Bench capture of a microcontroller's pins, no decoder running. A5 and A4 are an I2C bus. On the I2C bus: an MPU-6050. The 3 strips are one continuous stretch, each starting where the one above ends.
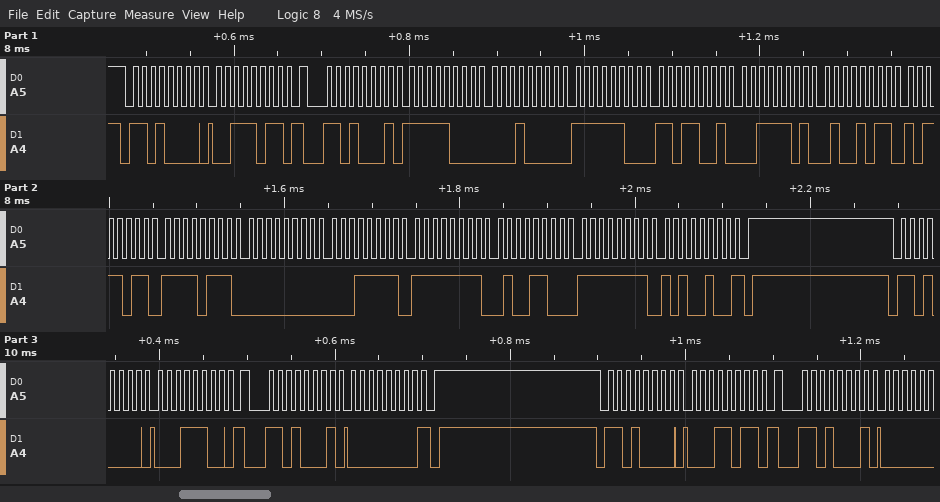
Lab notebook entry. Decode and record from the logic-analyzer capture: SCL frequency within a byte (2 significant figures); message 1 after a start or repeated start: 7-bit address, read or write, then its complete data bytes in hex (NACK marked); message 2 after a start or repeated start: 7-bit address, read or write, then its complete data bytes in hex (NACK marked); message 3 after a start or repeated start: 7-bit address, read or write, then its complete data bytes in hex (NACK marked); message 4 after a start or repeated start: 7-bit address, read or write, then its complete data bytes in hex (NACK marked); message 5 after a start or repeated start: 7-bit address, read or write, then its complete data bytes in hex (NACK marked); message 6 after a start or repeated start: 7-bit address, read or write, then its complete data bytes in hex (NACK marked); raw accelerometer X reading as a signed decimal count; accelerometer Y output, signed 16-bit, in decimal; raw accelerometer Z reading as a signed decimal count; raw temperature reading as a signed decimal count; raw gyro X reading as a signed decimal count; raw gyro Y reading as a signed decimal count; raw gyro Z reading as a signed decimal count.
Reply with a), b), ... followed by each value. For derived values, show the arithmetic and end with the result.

a) 100 kHz
b) 0x68 write: 3B
c) 0x68 read: F8 10 FC D9 3D 4B BB F7 00 1F FF 4C FF A4 NACK
d) 0x68 write: 1C
e) 0x68 read: 00 NACK
f) 0x68 write: 1B
g) 0x68 read
h) 0xF810 = -2032
i) 0xFCD9 = -807
j) 0x3D4B = 15691
k) 0xBBF7 = -17417
l) 0x001F = 31
m) 0xFF4C = -180
n) 0xFFA4 = -92
